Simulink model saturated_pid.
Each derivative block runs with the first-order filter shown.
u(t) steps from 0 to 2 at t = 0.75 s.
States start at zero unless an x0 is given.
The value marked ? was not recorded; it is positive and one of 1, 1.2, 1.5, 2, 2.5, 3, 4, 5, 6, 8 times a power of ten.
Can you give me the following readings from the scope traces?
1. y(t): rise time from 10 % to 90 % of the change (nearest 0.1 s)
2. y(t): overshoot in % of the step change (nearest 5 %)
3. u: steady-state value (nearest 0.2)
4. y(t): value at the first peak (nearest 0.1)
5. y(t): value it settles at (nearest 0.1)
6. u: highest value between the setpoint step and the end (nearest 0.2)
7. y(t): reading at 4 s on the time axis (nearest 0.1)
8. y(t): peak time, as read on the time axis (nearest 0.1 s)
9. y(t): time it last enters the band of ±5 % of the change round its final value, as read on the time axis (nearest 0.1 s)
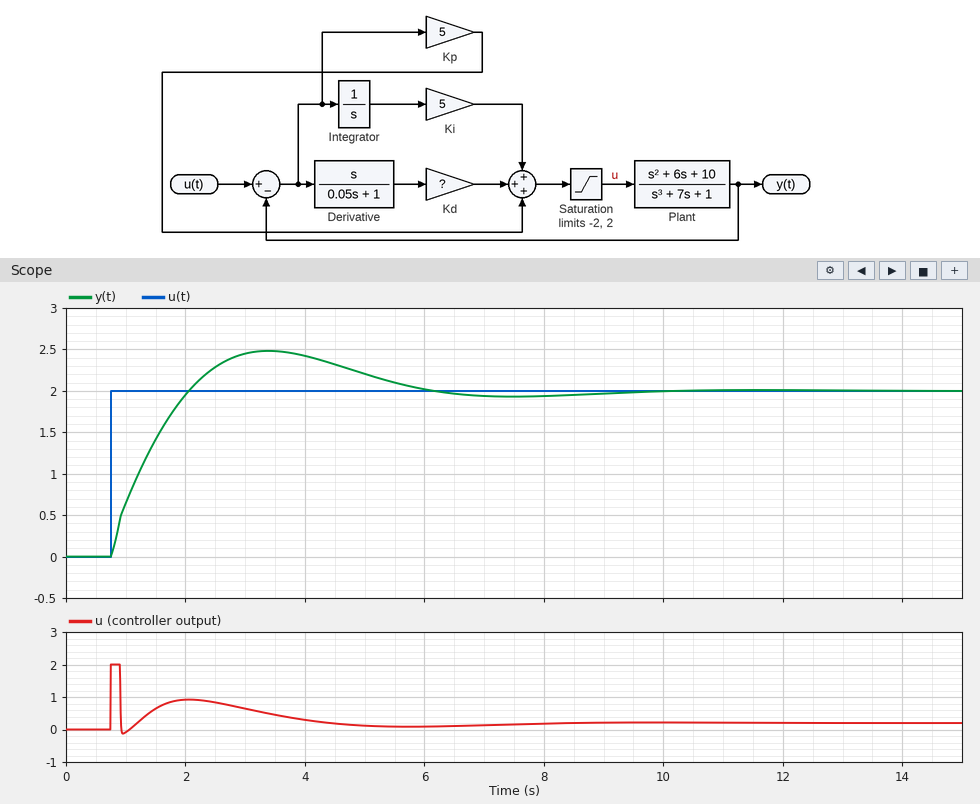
1.0 s
25 %
0.2
2.5
2.0
2.0
2.4
3.4 s
5.5 s
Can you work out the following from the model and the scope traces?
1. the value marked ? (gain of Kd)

5
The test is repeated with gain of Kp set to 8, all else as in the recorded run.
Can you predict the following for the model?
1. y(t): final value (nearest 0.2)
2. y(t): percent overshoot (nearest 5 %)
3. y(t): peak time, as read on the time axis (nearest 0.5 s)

2.0
15 %
3.0 s
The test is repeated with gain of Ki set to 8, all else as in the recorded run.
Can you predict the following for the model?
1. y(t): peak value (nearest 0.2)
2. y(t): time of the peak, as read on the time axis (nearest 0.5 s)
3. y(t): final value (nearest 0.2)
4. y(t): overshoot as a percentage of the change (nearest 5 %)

2.6
3.0 s
2.0
30 %
